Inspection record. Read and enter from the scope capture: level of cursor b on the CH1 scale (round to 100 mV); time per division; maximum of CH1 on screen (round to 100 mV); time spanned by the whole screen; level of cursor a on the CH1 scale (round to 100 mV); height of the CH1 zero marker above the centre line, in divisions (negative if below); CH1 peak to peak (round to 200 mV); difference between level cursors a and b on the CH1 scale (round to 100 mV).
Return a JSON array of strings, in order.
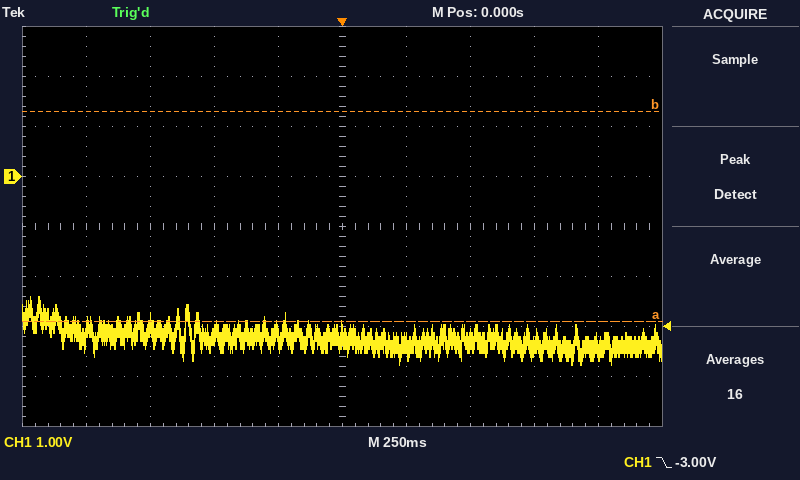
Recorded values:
["1.3 V", "250 ms", "-2.4 V", "2.5 s", "-2.9 V", "+1.0 div", "1.4 V", "4.2 V"]
